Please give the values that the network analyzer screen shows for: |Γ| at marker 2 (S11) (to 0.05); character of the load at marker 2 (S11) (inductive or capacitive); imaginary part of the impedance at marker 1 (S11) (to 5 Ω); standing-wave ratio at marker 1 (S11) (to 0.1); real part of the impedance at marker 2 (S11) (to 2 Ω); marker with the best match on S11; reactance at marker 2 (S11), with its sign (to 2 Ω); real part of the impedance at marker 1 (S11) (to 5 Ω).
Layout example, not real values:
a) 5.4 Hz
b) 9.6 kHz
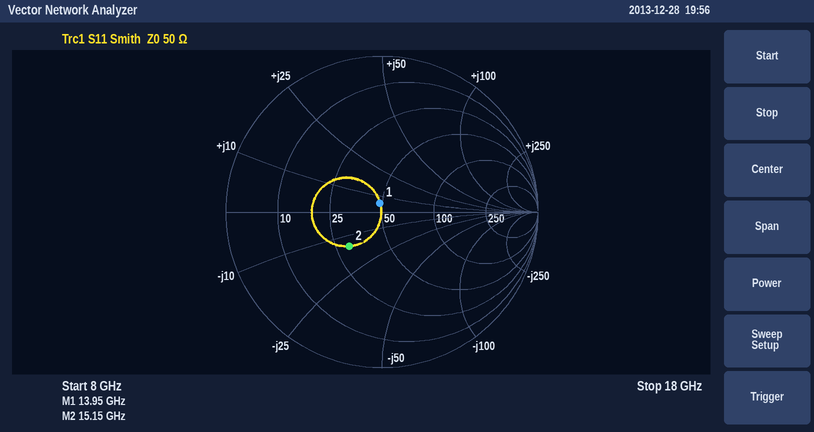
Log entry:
a) 0.30
b) capacitive
c) +5 Ω
d) 1.1
e) 30 Ω
f) marker 1
g) -14 Ω
h) 50 Ω
